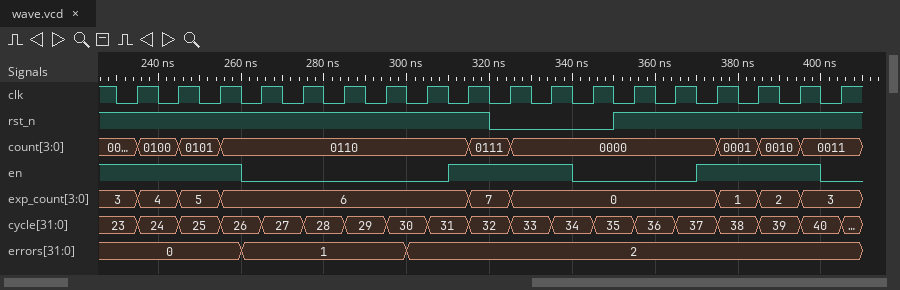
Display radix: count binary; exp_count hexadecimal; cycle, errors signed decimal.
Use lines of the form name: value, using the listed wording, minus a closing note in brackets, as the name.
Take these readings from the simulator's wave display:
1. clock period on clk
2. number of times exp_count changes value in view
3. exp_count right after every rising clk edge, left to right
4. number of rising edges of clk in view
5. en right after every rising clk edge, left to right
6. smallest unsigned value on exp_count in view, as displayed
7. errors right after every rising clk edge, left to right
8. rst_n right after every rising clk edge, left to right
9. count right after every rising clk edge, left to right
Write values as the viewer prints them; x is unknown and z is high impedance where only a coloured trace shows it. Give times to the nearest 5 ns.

clock period on clk: 10 ns
number of times exp_count changes value in view: 8
exp_count right after every rising clk edge, left to right: 4, 5, 6, 6, 6, 6, 6, 6, 7, 0, 0, 0, 0, 0, 1, 2, 3, 3
number of rising edges of clk in view: 18
en right after every rising clk edge, left to right: 1 1 1 0 0 0 0 0 1 1 1 0 0 0 1 1 1 0
smallest unsigned value on exp_count in view, as displayed: 0
errors right after every rising clk edge, left to right: 0, 0, 0, 1, 1, 1, 1, 2, 2, 2, 2, 2, 2, 2, 2, 2, 2, 2
rst_n right after every rising clk edge, left to right: 1 1 1 1 1 1 1 1 1 0 0 0 1 1 1 1 1 1
count right after every rising clk edge, left to right: 0100, 0101, 0110, 0110, 0110, 0110, 0110, 0110, 0111, 0000, 0000, 0000, 0000, 0000, 0001, 0010, 0011, 0011
